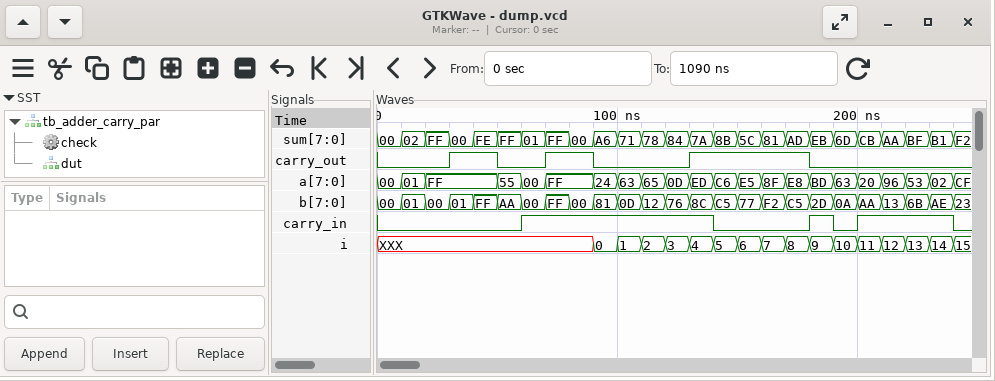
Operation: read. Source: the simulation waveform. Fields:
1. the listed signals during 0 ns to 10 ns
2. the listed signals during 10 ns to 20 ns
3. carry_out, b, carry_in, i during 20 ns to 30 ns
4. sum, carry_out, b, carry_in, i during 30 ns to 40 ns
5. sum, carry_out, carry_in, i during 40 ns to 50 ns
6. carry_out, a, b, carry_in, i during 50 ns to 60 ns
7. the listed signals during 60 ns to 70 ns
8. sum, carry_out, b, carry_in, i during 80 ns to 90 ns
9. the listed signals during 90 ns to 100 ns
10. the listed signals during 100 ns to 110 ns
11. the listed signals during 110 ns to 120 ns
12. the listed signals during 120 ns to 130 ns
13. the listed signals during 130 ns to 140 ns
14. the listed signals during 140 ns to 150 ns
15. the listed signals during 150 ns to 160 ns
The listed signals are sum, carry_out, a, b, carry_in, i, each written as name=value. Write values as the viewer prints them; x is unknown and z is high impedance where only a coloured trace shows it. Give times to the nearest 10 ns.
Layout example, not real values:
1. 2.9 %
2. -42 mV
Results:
1. sum=00, carry_out=0, a=00, b=00, carry_in=0, i=XXX
2. sum=02, carry_out=0, a=01, b=01, carry_in=0, i=XXX
3. carry_out=0, b=00, carry_in=0, i=XXX
4. sum=00, carry_out=1, b=01, carry_in=0, i=XXX
5. sum=FE, carry_out=1, carry_in=0, i=XXX
6. carry_out=0, a=55, b=AA, carry_in=0, i=XXX
7. sum=01, carry_out=0, a=00, b=00, carry_in=1, i=XXX
8. sum=00, carry_out=1, b=00, carry_in=1, i=XXX
9. sum=A6, carry_out=0, a=24, b=81, carry_in=1, i=0
10. sum=71, carry_out=0, a=63, b=0D, carry_in=1, i=1
11. sum=78, carry_out=0, a=65, b=12, carry_in=1, i=2
12. sum=84, carry_out=0, a=0D, b=76, carry_in=1, i=3
13. sum=7A, carry_out=1, a=ED, b=8C, carry_in=1, i=4
14. sum=8B, carry_out=1, a=C6, b=C5, carry_in=0, i=5
15. sum=5C, carry_out=1, a=E5, b=77, carry_in=0, i=6
